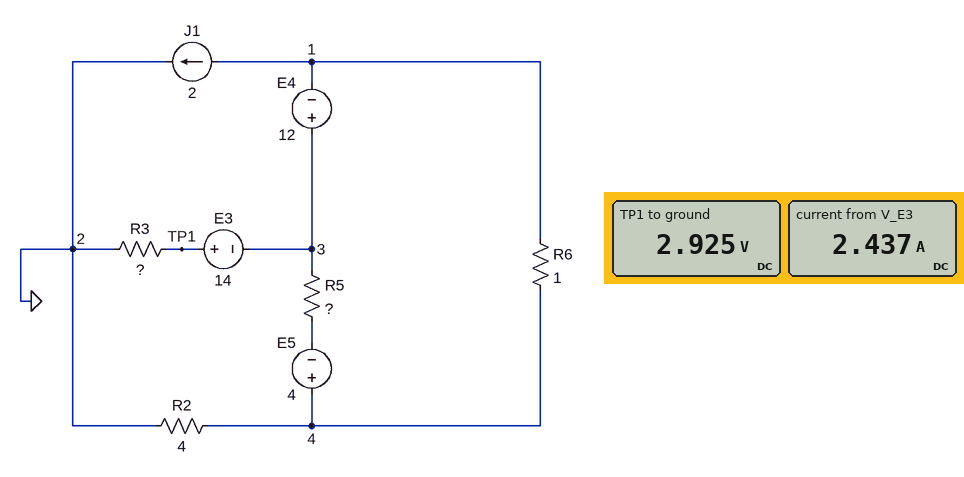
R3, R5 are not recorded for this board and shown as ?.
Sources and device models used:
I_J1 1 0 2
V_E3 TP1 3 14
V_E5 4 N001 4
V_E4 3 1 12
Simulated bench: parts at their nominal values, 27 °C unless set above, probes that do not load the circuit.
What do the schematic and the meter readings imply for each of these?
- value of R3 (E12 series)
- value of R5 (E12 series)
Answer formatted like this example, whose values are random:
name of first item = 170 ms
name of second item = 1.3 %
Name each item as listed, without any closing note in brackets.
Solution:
value of R3 = 1.2 Ω
value of R5 = 12 Ω
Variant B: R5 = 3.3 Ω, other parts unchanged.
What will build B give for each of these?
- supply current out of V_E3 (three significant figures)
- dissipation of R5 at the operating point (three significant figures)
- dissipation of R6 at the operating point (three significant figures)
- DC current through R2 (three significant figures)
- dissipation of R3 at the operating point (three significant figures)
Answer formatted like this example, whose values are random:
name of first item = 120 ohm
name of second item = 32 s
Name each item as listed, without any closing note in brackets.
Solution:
supply current out of V_E3 = 2.14 A
dissipation of R5 at the operating point = 25.1 W
dissipation of R6 at the operating point = 47.5 W
DC current through R2 = 4.14 A
dissipation of R3 at the operating point = 5.47 W
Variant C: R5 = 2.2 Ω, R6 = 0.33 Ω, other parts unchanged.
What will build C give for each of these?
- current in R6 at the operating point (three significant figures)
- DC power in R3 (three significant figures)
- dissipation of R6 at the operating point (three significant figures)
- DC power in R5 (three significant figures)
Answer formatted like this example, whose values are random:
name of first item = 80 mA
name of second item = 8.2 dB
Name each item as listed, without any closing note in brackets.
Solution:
current in R6 at the operating point = 10.5 A
DC power in R3 = 9.38 W
dissipation of R6 at the operating point = 36.3 W
DC power in R5 = 71.4 W
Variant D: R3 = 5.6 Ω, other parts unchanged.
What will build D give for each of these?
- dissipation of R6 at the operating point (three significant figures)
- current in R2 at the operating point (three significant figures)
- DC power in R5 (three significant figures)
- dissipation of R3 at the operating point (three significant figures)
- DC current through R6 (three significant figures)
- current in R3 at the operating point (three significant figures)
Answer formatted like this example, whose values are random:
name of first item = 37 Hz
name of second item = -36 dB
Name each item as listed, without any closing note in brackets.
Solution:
dissipation of R6 at the operating point = 19.2 W
current in R2 at the operating point = 3.42 A
DC power in R5 = 11.2 W
dissipation of R3 at the operating point = 11.3 W
DC current through R6 = 4.39 A
current in R3 at the operating point = 1.42 A
